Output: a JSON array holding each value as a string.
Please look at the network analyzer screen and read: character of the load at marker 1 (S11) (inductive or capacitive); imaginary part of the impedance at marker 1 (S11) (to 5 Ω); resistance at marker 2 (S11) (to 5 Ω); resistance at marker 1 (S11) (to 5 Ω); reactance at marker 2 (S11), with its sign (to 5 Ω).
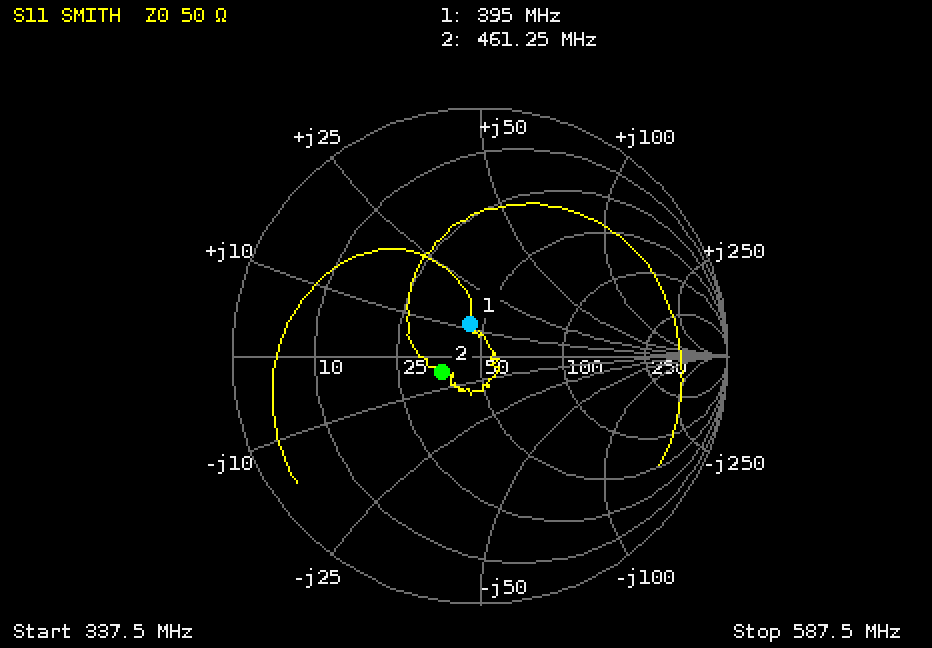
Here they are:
["inductive", "+10 Ω", "35 Ω", "45 Ω", "-5 Ω"]
